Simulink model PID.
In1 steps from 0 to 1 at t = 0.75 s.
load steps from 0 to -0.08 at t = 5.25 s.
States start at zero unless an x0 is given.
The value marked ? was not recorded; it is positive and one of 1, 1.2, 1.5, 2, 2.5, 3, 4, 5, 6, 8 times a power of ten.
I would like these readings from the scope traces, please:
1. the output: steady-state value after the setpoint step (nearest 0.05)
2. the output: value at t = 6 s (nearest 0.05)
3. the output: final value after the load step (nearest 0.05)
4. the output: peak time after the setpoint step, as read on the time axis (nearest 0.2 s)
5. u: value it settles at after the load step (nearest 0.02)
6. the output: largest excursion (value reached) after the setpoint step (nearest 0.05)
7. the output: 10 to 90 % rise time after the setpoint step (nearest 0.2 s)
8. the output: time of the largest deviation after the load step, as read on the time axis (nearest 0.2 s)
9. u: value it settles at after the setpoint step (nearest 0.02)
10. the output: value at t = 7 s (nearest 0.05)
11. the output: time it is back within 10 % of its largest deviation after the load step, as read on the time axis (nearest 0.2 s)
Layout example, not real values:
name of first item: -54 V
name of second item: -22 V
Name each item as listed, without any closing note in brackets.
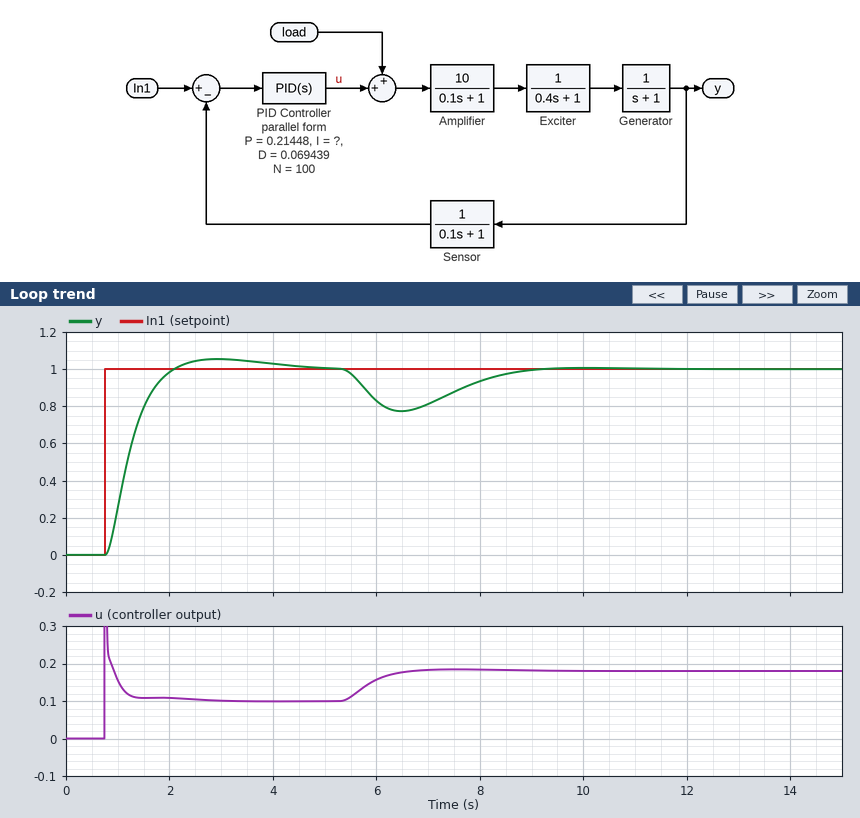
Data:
the output: steady-state value after the setpoint step: 1.00
the output: value at t = 6 s: 0.85
the output: final value after the load step: 1.00
the output: peak time after the setpoint step, as read on the time axis: 3.0 s
u: value it settles at after the load step: 0.18
the output: largest excursion (value reached) after the setpoint step: 1.05
the output: 10 to 90 % rise time after the setpoint step: 0.8 s
the output: time of the largest deviation after the load step, as read on the time axis: 6.4 s
u: value it settles at after the setpoint step: 0.10
the output: value at t = 7 s: 0.80
the output: time it is back within 10 % of its largest deviation after the load step, as read on the time axis: 8.6 s
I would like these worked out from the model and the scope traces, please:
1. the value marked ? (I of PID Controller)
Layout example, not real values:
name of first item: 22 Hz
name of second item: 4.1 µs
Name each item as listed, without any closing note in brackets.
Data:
the value marked ?: 0.2
